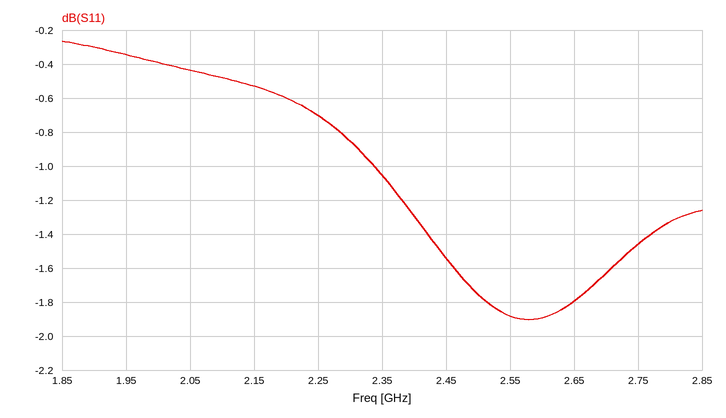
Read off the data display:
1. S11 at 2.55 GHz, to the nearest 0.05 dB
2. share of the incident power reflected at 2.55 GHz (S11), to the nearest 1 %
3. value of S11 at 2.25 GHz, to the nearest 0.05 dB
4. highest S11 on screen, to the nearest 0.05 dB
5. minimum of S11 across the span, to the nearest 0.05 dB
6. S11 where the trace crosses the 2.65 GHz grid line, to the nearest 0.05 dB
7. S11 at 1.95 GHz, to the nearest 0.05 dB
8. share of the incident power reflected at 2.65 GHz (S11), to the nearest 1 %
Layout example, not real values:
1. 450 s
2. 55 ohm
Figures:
1. -1.90 dB
2. 65 %
3. -0.70 dB
4. -0.25 dB
5. -1.90 dB
6. -1.80 dB
7. -0.35 dB
8. 66 %
